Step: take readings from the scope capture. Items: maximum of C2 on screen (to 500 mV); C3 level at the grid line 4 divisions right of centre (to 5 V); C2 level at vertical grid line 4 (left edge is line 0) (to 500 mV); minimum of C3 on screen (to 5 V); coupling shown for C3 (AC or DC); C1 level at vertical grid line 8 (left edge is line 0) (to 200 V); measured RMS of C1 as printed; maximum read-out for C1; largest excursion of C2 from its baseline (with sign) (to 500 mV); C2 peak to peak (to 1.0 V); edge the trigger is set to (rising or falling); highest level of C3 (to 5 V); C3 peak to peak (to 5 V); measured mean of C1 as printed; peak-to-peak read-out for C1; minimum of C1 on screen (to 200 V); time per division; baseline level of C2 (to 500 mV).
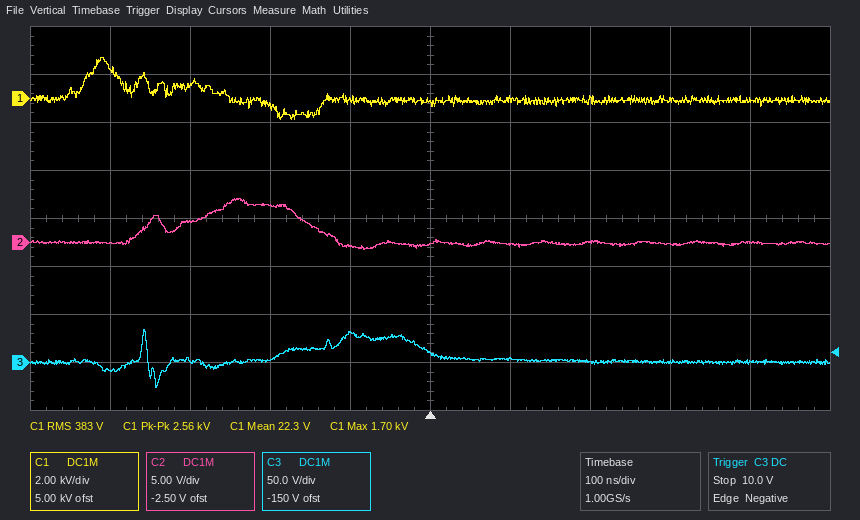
4.5 V
0 V
-500 mV
-25 V
DC
0.0 kV
383 V
1.70 kV
+4.5 V
5.0 V
falling
35 V
60 V
22.3 V
2.56 kV
-800 V
100 ns
0.0 V
